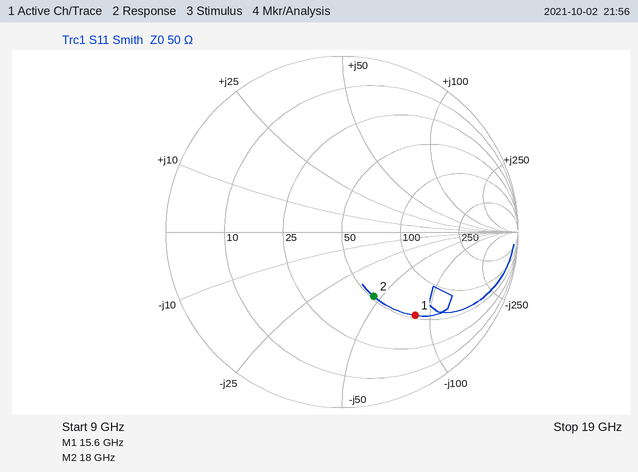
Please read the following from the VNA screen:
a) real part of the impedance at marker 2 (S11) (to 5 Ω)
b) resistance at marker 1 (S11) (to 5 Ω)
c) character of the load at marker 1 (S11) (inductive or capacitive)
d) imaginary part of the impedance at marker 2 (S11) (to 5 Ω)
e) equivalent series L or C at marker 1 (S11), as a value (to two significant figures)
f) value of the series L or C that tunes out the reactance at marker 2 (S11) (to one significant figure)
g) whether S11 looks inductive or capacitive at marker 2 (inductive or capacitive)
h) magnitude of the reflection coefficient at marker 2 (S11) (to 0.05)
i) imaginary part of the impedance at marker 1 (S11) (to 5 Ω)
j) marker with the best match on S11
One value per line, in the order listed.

50 Ω
55 Ω
capacitive
-45 Ω
120 fF
400 pH
capacitive
0.40
-85 Ω
marker 2
